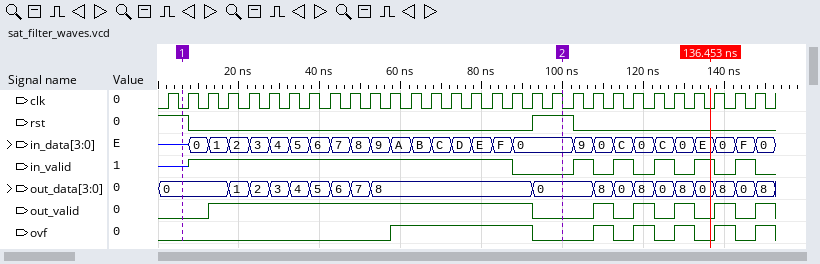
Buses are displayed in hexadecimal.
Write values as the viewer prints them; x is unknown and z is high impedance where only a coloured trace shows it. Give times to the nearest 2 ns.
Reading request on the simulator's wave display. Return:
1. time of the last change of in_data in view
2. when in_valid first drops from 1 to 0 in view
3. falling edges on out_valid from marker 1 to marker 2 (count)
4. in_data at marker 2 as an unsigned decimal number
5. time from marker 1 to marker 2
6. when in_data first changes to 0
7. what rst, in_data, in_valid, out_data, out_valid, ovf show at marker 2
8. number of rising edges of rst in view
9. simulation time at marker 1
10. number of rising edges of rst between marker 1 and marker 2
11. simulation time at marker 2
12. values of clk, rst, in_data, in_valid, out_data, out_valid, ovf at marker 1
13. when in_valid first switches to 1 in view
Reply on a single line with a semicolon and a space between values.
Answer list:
148 ns; 88 ns; 1; 0; 94 ns; 8 ns; rst=1, in_data=0, in_valid=0, out_data=0, out_valid=0, ovf=0; 1; 6 ns; 1; 100 ns; clk=0, rst=1, in_data=z, in_valid=z, out_data=0, out_valid=0, ovf=0; 8 ns
